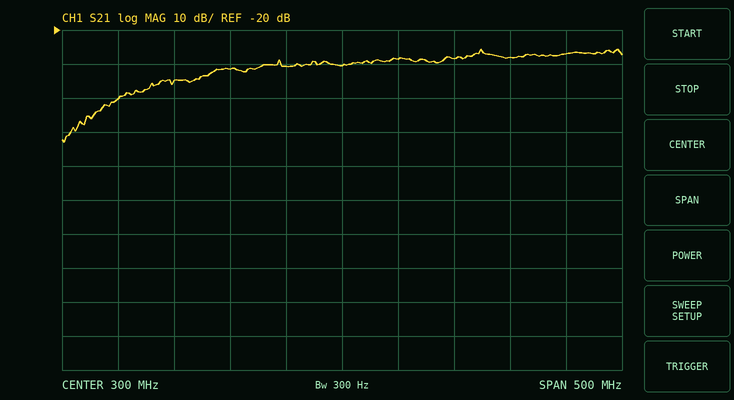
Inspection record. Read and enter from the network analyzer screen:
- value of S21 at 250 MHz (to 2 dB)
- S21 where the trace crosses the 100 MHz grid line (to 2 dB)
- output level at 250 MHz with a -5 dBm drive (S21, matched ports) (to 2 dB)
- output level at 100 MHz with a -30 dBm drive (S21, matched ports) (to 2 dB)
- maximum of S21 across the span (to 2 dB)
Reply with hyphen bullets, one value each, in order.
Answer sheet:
- -30 dB
- -40 dB
- -36 dBm
- -70 dBm
- -26 dB
